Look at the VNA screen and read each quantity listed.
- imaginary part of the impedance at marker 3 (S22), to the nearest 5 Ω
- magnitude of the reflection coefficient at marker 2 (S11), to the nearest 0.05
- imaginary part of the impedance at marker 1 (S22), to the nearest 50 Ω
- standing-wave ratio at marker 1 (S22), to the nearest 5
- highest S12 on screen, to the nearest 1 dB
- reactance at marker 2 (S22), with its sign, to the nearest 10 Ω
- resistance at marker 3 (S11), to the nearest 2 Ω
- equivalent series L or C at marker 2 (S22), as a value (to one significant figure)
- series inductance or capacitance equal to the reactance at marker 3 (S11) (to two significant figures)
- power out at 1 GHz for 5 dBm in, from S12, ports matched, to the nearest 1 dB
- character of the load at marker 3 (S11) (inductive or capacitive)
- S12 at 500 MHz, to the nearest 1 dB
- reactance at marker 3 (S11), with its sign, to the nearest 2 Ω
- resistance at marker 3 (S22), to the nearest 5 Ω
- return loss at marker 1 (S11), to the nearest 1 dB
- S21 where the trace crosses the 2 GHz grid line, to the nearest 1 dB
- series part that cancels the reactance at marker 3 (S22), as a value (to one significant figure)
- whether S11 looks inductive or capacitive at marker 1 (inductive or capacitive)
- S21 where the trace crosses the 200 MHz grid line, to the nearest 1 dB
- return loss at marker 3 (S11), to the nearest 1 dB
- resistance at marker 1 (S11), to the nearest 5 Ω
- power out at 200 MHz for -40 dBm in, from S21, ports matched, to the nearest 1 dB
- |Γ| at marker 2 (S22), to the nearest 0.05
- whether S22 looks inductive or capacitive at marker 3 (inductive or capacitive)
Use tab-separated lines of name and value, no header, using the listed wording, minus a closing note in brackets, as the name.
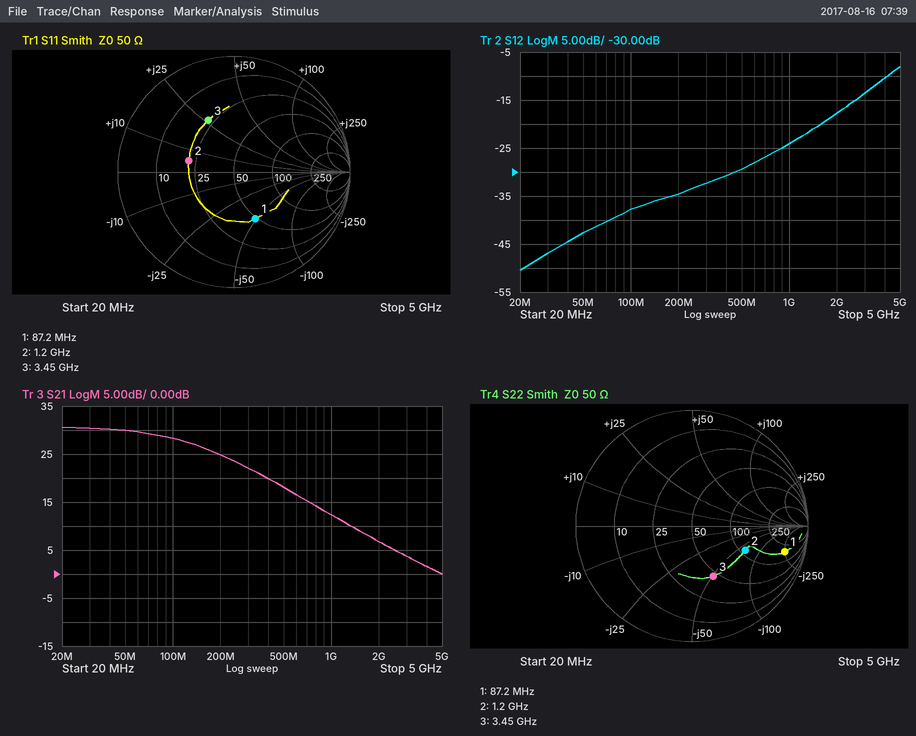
imaginary part of the impedance at marker 3 (S22), to the nearest 5 Ω	-50 Ω
magnitude of the reflection coefficient at marker 2 (S11), to the nearest 0.05	0.40
imaginary part of the impedance at marker 1 (S22), to the nearest 50 Ω	-250 Ω
standing-wave ratio at marker 1 (S22), to the nearest 5	10
highest S12 on screen, to the nearest 1 dB	-8 dB
reactance at marker 2 (S22), with its sign, to the nearest 10 Ω	-60 Ω
resistance at marker 3 (S11), to the nearest 2 Ω	22 Ω
equivalent series L or C at marker 2 (S22), as a value	2 pF
series inductance or capacitance equal to the reactance at marker 3 (S11)	1.2 nH
power out at 1 GHz for 5 dBm in, from S12, ports matched, to the nearest 1 dB	-19 dBm
character of the load at marker 3 (S11)	inductive
S12 at 500 MHz, to the nearest 1 dB	-29 dB
reactance at marker 3 (S11), with its sign, to the nearest 2 Ω	+26 Ω
resistance at marker 3 (S22), to the nearest 5 Ω	45 Ω
return loss at marker 1 (S11), to the nearest 1 dB	7 dB
S21 where the trace crosses the 2 GHz grid line, to the nearest 1 dB	7 dB
series part that cancels the reactance at marker 3 (S22), as a value	2 nH
whether S11 looks inductive or capacitive at marker 1	capacitive
S21 where the trace crosses the 200 MHz grid line, to the nearest 1 dB	25 dB
return loss at marker 3 (S11), to the nearest 1 dB	6 dB
resistance at marker 1 (S11), to the nearest 5 Ω	50 Ω
power out at 200 MHz for -40 dBm in, from S21, ports matched, to the nearest 1 dB	-15 dBm
|Γ| at marker 2 (S22), to the nearest 0.05	0.50
whether S22 looks inductive or capacitive at marker 3	capacitive
